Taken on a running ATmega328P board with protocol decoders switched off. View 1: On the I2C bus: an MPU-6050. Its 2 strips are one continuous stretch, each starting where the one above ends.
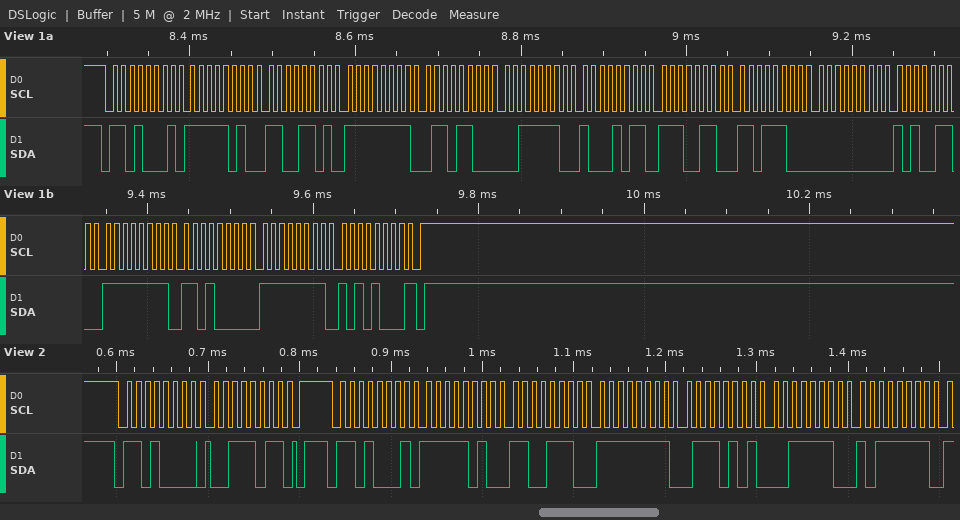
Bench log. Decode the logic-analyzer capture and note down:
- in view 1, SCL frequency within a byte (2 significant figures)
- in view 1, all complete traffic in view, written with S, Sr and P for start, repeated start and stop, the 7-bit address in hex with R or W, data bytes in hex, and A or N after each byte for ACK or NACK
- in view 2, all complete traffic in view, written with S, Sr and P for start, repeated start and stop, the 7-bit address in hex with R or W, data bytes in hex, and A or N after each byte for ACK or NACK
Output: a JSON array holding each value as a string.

["100 kHz", "S 68R A FA A CD A FF A 6C A 3E A 8B A E6 A DC A 00 A A6 A FF A D0 A FF A A8 N P", "S 68W A 3B A P S 68R A FA A CE A FF A 75 A 3E A BF A"]
